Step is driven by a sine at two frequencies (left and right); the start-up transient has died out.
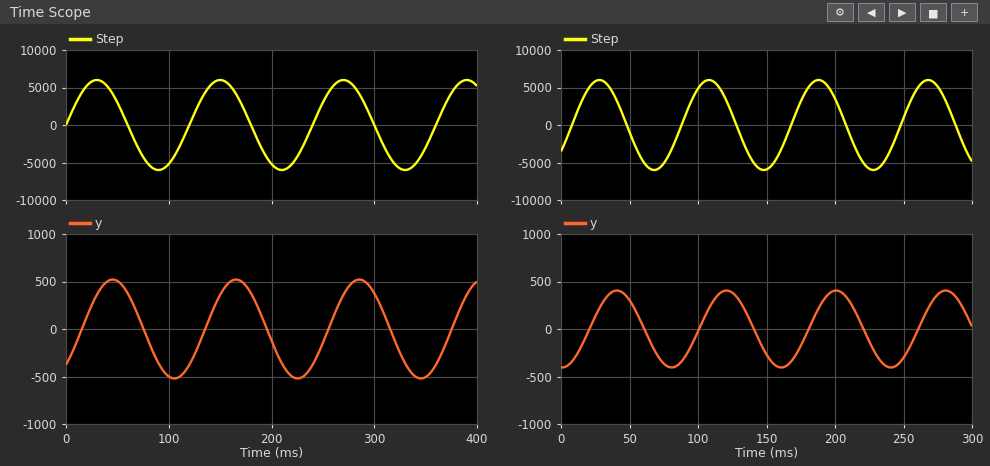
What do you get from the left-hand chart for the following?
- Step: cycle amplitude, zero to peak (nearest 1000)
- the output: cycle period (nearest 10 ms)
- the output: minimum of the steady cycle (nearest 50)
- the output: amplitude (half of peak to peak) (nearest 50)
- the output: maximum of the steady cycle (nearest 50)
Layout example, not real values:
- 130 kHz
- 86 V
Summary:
- 6000
- 120 ms
- -500
- 500
- 500
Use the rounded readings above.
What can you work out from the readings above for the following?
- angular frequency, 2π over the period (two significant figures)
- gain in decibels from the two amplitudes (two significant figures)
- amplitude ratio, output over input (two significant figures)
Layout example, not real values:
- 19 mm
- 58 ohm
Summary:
- 0.052 rad/ms
- -22 dB
- 0.083
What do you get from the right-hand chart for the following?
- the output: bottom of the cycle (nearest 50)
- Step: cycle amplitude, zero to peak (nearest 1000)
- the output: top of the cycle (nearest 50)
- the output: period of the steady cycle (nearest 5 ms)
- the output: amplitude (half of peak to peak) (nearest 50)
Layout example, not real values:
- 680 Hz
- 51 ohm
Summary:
- -400
- 6000
- 400
- 80 ms
- 400
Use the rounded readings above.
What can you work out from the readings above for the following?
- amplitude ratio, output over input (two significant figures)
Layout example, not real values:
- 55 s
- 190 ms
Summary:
- 0.067
